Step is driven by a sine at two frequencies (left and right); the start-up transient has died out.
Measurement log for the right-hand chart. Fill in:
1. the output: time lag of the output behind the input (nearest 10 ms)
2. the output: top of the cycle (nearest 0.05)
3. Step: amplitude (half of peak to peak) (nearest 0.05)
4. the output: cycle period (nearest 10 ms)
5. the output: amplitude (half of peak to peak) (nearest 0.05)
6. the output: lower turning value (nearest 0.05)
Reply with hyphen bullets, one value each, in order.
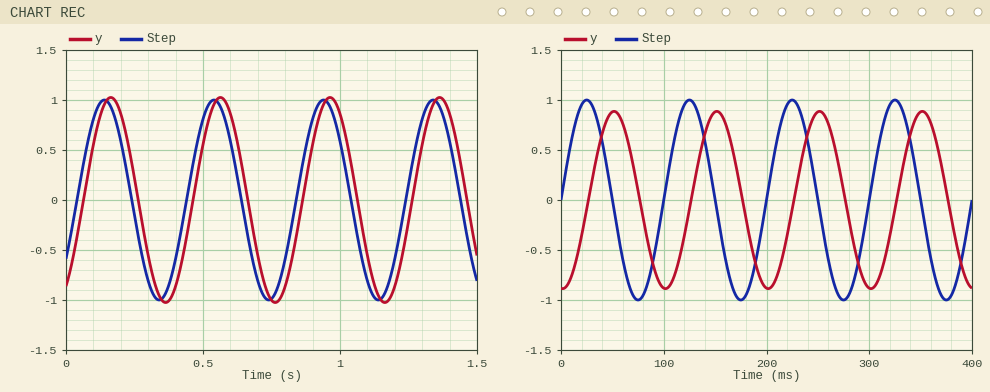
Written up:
- 30 ms
- 0.90
- 1.00
- 100 ms
- 0.90
- -0.90
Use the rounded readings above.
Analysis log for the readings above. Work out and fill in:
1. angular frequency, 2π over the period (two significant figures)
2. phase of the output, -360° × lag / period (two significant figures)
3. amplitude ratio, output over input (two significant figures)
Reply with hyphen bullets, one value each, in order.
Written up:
- 0.063 rad/ms
- -110°
- 0.90
